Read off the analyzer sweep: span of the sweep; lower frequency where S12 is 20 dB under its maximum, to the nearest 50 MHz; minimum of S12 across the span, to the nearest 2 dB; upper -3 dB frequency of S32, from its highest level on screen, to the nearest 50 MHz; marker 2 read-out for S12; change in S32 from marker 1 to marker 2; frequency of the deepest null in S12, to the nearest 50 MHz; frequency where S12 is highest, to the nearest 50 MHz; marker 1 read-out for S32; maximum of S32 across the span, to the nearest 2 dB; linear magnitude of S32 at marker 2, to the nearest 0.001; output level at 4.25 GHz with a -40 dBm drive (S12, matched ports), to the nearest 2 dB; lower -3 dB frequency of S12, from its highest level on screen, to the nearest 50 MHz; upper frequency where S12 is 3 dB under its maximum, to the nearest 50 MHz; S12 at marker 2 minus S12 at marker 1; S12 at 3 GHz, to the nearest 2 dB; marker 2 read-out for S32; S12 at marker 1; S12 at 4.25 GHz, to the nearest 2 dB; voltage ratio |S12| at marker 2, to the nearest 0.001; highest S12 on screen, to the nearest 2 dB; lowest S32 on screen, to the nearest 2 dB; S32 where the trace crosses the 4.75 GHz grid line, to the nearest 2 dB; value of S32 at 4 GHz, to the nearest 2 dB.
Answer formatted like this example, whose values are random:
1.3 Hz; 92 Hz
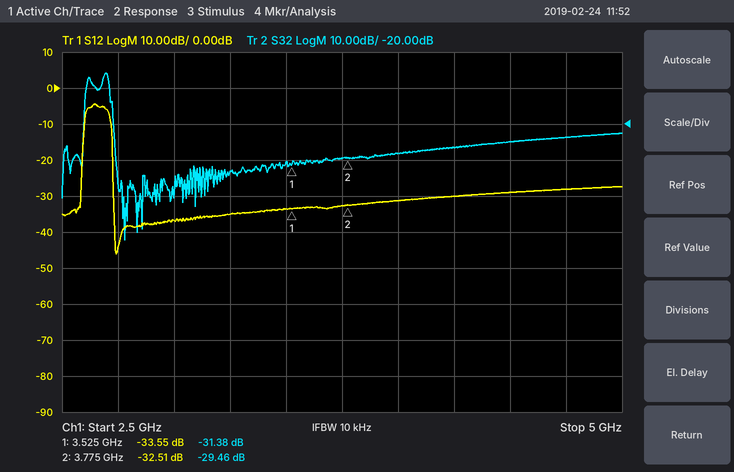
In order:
2.5 GHz; 2.60 GHz; -46 dB; 2.70 GHz; -32.51 dB; 1.92 dB; 2.75 GHz; 2.65 GHz; -31.38 dB; -6 dB; 0.034; -70 dBm; 2.60 GHz; 2.70 GHz; 1.04 dB; -36 dB; -29.46 dB; -33.55 dB; -30 dB; 0.024; -4 dB; -52 dB; -24 dB; -28 dB
